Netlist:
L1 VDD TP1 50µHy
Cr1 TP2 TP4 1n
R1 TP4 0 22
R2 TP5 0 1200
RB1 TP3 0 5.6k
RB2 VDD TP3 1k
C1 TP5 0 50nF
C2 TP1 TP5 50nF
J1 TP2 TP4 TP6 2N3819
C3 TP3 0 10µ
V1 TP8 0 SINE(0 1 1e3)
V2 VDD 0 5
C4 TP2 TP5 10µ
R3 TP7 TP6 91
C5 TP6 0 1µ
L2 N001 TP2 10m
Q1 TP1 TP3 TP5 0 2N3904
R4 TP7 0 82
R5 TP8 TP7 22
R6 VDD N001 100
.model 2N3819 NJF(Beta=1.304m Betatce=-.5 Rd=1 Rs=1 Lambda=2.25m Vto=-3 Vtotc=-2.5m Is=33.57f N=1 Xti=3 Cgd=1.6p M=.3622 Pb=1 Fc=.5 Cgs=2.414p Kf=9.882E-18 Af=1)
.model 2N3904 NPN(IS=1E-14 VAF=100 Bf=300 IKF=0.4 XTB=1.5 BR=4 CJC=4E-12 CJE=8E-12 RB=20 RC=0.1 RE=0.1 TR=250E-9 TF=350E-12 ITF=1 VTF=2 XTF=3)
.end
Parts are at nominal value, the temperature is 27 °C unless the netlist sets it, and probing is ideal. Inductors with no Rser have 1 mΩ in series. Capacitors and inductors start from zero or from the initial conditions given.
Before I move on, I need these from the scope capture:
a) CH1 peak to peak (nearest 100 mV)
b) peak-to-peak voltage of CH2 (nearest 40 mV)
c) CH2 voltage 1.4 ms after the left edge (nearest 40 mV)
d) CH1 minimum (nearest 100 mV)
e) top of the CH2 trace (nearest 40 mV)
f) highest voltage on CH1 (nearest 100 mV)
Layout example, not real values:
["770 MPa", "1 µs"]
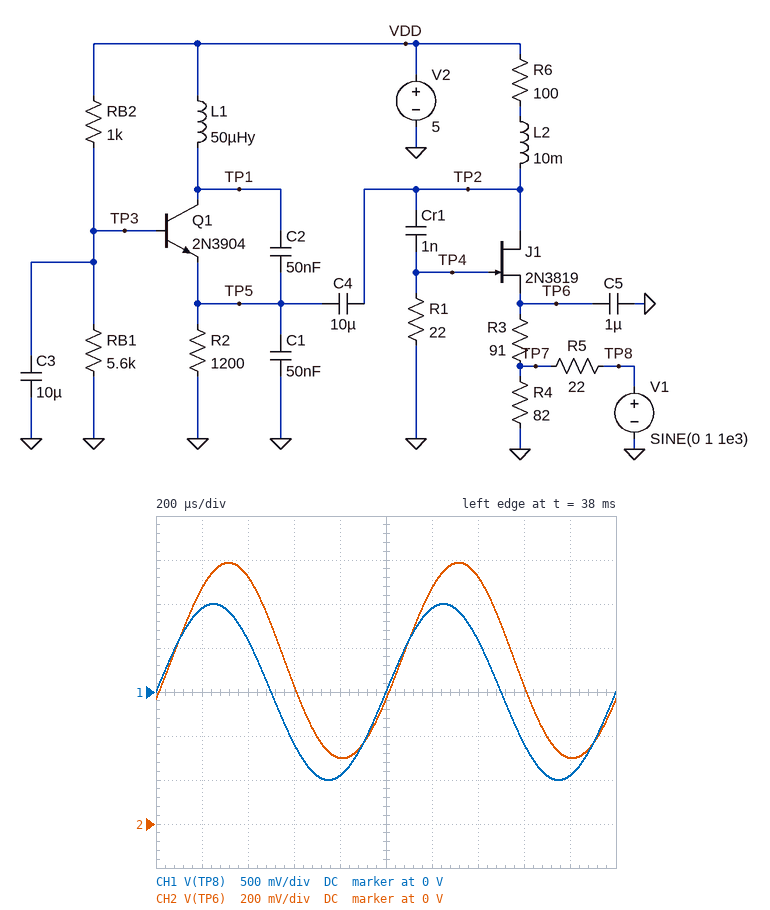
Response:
["2.0 V", "880 mV", "1.12 V", "-1.0 V", "1.20 V", "1.0 V"]
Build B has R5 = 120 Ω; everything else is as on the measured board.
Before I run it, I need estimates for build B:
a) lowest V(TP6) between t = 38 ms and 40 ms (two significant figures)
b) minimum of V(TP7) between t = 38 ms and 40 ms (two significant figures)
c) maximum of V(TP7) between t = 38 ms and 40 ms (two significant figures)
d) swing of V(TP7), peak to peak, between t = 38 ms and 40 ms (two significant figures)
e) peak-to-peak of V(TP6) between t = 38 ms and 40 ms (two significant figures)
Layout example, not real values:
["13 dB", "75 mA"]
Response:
["650 mV", "-34 mV", "630 mV", "660 mV", "410 mV"]
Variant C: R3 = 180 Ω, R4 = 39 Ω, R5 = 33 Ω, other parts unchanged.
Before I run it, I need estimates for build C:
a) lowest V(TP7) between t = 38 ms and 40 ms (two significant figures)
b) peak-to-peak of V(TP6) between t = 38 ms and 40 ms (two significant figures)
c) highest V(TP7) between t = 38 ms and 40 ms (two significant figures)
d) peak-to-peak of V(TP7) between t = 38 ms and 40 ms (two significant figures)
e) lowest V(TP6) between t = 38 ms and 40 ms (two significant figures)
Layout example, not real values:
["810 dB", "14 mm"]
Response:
["-420 mV", "460 mV", "600 mV", "1.0 V", "790 mV"]
